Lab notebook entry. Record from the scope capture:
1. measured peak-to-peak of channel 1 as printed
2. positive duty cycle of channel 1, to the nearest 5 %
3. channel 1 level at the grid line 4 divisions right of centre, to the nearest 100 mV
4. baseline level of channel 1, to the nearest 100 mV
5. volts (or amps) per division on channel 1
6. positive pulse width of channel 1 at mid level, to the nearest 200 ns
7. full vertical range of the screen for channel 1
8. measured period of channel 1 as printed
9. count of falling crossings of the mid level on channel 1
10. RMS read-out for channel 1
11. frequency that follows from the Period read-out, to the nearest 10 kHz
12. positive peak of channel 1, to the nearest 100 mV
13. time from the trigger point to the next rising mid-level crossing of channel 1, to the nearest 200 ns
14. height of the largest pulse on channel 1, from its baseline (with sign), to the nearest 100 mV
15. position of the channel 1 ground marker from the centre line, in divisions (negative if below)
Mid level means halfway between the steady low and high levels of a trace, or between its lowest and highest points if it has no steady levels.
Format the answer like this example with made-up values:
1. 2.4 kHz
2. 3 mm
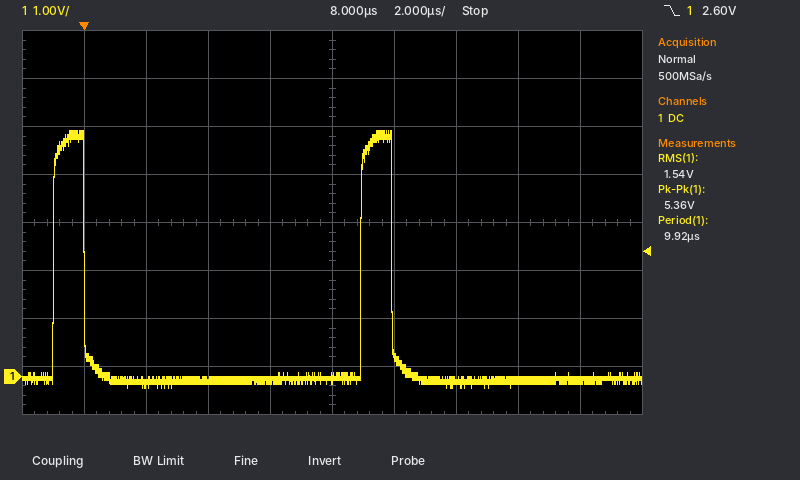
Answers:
1. 5.36 V
2. 10 %
3. -100 mV
4. -100 mV
5. 1 V
6. 1.0 µs
7. 8 V
8. 9.92 µs
9. 2
10. 1.54 V
11. 100 kHz
12. 5.1 V
13. 9.0 µs
14. +5.2 V
15. -3.2 div
